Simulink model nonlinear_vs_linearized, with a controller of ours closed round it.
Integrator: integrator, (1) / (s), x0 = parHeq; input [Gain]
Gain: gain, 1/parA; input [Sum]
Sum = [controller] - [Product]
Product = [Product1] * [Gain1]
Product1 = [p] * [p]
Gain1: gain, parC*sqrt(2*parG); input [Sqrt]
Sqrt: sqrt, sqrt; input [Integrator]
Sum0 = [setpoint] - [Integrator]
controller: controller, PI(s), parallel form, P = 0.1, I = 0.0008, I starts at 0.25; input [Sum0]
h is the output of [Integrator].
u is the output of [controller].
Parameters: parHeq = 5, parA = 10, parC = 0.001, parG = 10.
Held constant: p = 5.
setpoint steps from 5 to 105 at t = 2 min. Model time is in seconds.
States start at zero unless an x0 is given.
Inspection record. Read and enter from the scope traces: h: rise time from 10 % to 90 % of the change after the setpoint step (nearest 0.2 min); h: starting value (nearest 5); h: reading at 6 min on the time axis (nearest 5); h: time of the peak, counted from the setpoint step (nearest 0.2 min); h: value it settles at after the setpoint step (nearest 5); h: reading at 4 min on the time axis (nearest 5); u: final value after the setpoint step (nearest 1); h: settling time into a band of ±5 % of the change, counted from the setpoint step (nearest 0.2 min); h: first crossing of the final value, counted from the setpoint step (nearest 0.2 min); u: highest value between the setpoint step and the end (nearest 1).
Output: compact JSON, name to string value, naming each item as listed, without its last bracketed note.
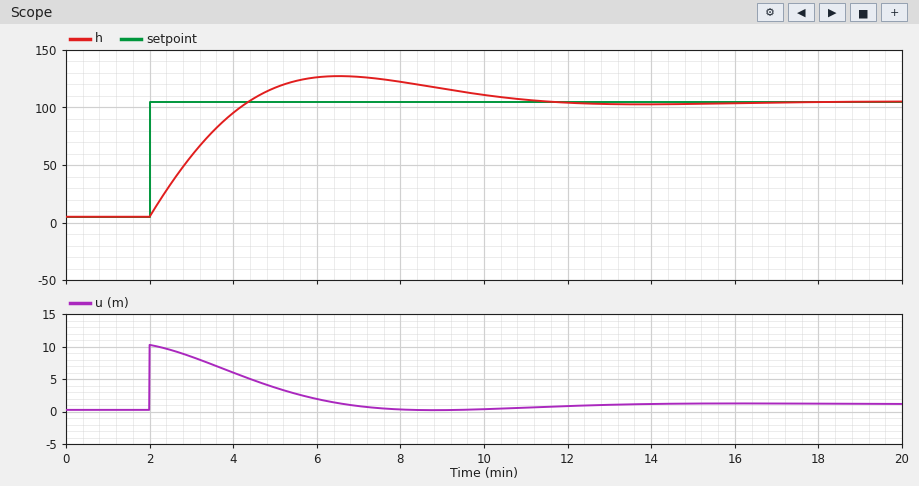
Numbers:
{"h: rise time from 10 % to 90 % of the change after the setpoint step": "1.8 min", "h: starting value": "5", "h: reading at 6 min on the time axis": "125", "h: time of the peak, counted from the setpoint step": "4.6 min", "h: value it settles at after the setpoint step": "105", "h: reading at 4 min on the time axis": "95", "u: final value after the setpoint step": "1", "h: settling time into a band of ±5 % of the change, counted from the setpoint step": "8.2 min", "h: first crossing of the final value, counted from the setpoint step": "2.4 min", "u: highest value between the setpoint step and the end": "10"}
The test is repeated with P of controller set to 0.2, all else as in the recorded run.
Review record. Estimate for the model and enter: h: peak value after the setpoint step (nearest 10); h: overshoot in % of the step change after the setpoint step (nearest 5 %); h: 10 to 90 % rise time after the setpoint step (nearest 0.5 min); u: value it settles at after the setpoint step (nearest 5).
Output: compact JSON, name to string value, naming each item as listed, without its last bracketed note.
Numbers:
{"h: peak value after the setpoint step": "110", "h: overshoot in % of the step change after the setpoint step": "10 %", "h: 10 to 90 % rise time after the setpoint step": "1.5 min", "u: value it settles at after the setpoint step": "0"}
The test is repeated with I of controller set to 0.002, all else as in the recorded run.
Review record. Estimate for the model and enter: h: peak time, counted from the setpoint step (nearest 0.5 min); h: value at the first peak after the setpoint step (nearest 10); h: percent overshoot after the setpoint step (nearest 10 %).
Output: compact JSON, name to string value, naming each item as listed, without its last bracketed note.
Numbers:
{"h: peak time, counted from the setpoint step": "3.0 min", "h: value at the first peak after the setpoint step": "140", "h: percent overshoot after the setpoint step": "40 %"}
